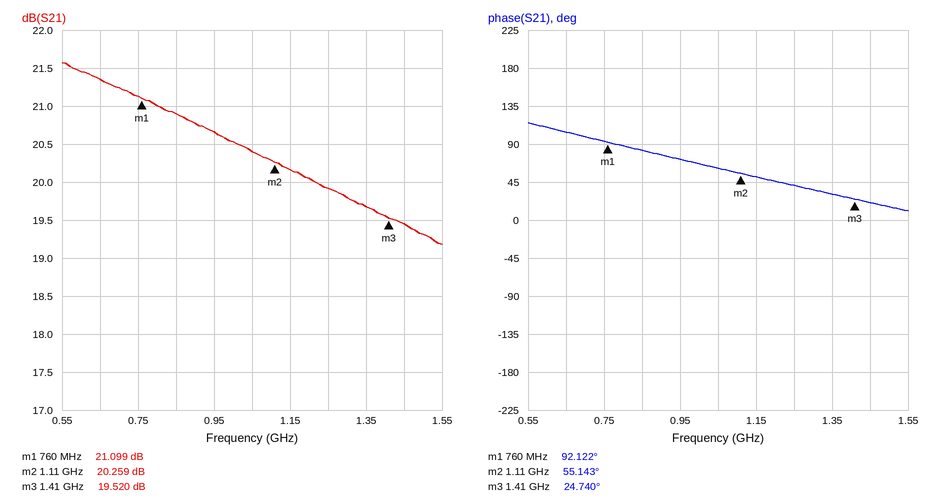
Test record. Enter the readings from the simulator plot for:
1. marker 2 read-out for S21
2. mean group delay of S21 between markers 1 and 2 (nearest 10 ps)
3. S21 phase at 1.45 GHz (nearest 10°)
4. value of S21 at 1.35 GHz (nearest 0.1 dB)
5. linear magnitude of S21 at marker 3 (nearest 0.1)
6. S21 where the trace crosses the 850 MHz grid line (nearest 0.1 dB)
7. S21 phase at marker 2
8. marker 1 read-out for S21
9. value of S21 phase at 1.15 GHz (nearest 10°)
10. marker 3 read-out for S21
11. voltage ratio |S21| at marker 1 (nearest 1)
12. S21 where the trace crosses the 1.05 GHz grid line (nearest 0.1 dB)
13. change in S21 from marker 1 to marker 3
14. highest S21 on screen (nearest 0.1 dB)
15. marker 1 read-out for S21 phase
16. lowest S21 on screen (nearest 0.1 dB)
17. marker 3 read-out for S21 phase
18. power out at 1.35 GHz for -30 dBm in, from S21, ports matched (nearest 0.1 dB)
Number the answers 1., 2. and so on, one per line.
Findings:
1. 20.259 dB
2. 290 ps
3. 20°
4. 19.7 dB
5. 9.5
6. 20.9 dB
7. 55.143°
8. 21.099 dB
9. 50°
10. 19.520 dB
11. 11
12. 20.4 dB
13. -1.579 dB
14. 21.6 dB
15. 92.122°
16. 19.2 dB
17. 24.740°
18. -10.3 dBm
